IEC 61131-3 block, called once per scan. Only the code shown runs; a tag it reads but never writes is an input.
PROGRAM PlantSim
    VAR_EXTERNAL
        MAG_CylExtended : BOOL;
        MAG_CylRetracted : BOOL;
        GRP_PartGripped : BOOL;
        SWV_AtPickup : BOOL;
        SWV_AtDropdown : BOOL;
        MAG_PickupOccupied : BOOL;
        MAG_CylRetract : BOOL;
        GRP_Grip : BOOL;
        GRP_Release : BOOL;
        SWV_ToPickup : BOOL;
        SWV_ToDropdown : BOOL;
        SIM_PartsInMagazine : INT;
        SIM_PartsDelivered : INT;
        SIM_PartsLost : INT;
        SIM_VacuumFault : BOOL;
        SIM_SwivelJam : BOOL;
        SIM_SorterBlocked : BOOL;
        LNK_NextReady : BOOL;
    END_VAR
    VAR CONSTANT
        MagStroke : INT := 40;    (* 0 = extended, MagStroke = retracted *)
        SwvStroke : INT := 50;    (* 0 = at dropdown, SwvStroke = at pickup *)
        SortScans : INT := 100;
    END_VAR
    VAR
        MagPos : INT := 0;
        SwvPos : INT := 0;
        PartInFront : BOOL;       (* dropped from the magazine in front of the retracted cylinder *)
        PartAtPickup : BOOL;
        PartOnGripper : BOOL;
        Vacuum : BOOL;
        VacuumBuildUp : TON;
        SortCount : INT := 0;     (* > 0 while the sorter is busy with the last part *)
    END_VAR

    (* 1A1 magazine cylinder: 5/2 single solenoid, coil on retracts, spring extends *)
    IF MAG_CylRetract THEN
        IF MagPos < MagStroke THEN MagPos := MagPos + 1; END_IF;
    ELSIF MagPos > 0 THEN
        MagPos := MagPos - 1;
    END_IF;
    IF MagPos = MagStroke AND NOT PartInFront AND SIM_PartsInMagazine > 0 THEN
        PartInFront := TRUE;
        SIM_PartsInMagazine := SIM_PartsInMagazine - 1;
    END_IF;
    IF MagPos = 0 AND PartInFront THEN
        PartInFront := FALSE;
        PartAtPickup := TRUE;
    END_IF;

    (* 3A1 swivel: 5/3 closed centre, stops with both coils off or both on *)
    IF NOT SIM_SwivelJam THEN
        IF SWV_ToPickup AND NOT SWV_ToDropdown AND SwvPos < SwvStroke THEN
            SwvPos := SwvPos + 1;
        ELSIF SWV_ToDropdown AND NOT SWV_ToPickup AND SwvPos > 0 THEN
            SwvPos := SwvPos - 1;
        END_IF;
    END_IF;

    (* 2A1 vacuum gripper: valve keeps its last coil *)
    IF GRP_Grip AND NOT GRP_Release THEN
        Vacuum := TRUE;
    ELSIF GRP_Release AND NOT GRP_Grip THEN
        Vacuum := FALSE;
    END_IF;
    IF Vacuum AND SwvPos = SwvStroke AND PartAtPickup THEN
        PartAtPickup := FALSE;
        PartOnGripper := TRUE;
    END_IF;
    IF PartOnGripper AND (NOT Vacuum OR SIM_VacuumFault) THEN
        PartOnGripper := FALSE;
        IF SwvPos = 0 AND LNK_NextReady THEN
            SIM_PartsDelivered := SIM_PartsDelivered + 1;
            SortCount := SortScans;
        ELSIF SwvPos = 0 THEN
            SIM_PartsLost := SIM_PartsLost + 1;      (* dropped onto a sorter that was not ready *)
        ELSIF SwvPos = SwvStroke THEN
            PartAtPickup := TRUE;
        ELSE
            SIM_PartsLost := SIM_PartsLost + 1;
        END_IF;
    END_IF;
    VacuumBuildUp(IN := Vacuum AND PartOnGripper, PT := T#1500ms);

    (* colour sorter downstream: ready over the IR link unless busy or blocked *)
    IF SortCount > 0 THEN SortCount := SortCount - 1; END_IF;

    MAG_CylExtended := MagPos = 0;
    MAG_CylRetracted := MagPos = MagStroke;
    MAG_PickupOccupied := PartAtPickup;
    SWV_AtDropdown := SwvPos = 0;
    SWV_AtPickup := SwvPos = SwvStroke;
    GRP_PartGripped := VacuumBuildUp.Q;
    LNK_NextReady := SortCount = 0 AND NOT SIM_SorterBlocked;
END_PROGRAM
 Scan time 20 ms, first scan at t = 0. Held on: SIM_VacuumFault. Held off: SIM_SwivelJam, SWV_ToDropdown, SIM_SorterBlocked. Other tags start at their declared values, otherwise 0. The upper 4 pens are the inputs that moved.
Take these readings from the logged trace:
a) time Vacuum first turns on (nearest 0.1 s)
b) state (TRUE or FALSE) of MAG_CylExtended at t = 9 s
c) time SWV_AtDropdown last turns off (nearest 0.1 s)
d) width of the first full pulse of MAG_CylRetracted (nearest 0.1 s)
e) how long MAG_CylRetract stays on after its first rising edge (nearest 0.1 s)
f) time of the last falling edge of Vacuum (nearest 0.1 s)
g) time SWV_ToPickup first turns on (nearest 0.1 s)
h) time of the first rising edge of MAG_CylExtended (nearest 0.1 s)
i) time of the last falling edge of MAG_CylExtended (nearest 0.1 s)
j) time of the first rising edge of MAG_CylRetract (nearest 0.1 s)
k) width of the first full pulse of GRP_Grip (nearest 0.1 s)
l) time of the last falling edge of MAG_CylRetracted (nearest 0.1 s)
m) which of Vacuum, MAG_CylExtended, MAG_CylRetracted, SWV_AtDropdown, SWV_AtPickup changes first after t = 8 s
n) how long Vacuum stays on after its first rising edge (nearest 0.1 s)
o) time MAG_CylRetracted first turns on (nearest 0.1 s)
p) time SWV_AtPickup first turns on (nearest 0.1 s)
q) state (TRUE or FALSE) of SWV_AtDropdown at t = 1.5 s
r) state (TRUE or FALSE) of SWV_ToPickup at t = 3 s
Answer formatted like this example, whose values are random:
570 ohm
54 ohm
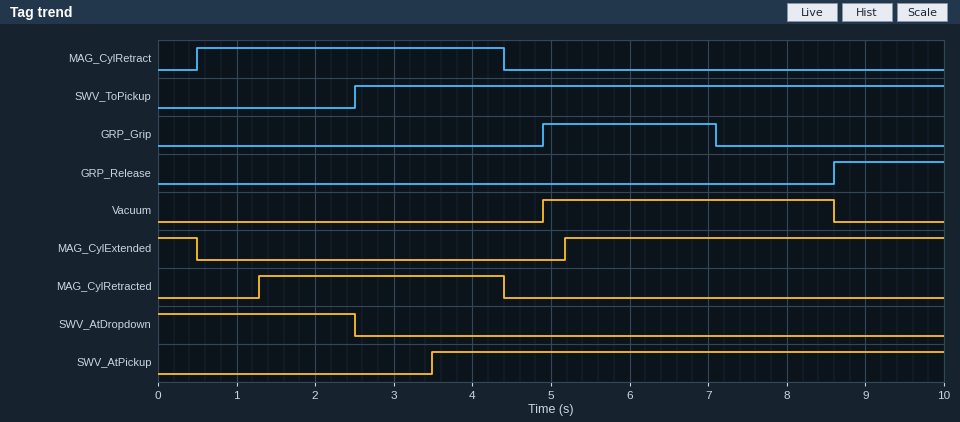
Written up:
4.9 s
TRUE
2.5 s
3.1 s
3.9 s
8.6 s
2.5 s
5.2 s
0.5 s
0.5 s
2.2 s
4.4 s
Vacuum
3.7 s
1.3 s
3.5 s
TRUE
TRUE
